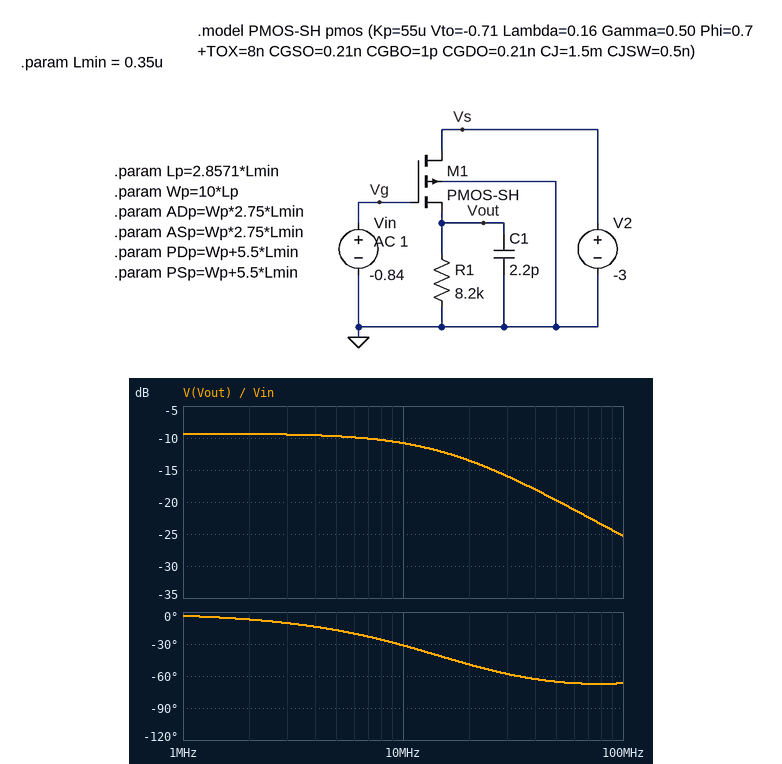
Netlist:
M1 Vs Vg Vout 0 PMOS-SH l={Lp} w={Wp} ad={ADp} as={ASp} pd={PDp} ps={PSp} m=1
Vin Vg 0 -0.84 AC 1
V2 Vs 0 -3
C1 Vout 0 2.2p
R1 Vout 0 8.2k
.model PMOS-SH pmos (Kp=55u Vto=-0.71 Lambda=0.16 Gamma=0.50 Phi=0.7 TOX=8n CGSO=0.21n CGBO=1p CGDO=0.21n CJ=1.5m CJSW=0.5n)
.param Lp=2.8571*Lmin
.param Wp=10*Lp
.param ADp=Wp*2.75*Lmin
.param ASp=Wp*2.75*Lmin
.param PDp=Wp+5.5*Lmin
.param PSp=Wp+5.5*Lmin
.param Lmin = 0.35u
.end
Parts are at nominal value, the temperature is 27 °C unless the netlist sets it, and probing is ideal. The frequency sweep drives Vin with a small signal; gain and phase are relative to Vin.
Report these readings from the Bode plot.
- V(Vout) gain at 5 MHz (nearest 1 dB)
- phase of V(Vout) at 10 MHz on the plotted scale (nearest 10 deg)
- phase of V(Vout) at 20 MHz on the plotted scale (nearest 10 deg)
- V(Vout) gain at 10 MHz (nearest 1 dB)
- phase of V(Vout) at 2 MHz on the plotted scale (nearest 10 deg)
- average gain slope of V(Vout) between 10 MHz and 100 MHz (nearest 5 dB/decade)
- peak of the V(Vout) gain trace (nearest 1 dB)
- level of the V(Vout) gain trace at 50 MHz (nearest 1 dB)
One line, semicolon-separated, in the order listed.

-10 dB; -30 deg; -50 deg; -11 dB; -10 deg; -15 dB/decade; -9 dB; -20 dB
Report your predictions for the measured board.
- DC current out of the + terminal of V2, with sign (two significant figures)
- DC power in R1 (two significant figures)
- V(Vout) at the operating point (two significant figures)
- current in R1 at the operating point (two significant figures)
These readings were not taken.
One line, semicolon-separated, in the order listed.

-3.5 µA; 100 nW; -29 mV; 3.5 µA
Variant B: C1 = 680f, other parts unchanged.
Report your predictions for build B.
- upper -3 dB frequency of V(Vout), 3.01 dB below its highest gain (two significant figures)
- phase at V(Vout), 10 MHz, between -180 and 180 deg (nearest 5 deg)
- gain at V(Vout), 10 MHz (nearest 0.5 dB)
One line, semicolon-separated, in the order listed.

49 MHz; -10 deg; -9.5 dB
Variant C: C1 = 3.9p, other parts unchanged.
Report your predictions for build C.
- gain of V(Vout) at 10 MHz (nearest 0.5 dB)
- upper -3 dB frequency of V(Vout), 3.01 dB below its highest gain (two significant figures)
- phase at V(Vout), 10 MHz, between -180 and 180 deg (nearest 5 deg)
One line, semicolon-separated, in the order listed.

-13.0 dB; 8.9 MHz; -45 deg
